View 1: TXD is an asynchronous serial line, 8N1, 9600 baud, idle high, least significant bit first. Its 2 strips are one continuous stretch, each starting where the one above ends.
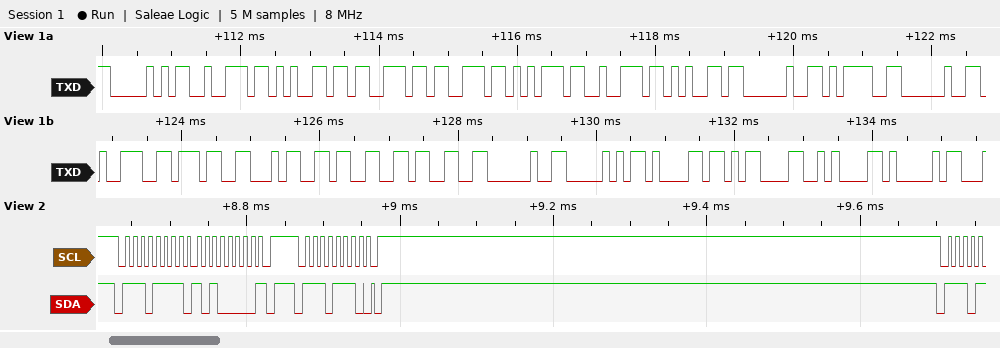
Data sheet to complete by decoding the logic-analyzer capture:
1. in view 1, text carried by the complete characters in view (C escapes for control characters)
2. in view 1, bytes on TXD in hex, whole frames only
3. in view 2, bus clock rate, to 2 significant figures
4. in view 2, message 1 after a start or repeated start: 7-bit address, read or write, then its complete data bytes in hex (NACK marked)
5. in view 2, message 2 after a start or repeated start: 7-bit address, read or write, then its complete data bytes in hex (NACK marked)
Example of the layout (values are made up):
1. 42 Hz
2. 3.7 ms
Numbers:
1. "Pressure = 97433 Pa\r\nA"
2. 50 72 65 73 73 75 72 65 20 3D 20 39 37 34 33 33 20 50 61 0D 0A 41
3. 100 kHz
4. 0x77 read: A0 NACK
5. 0x77 write
